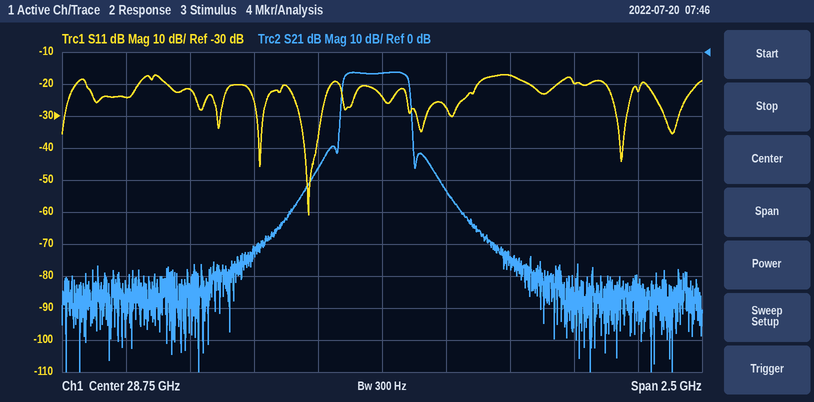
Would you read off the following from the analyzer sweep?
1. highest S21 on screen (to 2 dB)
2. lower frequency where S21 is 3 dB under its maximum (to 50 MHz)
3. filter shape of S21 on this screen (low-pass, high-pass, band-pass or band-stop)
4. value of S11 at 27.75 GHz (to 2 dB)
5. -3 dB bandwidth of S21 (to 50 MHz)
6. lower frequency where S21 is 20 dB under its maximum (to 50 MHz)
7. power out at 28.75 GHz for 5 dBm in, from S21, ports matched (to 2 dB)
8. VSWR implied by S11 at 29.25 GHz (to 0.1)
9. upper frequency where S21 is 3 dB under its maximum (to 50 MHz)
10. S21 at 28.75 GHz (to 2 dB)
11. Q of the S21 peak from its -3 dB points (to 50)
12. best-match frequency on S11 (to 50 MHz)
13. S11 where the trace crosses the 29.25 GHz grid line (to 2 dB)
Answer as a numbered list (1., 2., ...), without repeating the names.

1. -6 dB
2. 28.60 GHz
3. band-pass
4. -24 dB
5. 250 MHz
6. 28.60 GHz
7. -2 dBm
8. 1.3
9. 28.85 GHz
10. -6 dB
11. 100
12. 28.45 GHz
13. -18 dB
